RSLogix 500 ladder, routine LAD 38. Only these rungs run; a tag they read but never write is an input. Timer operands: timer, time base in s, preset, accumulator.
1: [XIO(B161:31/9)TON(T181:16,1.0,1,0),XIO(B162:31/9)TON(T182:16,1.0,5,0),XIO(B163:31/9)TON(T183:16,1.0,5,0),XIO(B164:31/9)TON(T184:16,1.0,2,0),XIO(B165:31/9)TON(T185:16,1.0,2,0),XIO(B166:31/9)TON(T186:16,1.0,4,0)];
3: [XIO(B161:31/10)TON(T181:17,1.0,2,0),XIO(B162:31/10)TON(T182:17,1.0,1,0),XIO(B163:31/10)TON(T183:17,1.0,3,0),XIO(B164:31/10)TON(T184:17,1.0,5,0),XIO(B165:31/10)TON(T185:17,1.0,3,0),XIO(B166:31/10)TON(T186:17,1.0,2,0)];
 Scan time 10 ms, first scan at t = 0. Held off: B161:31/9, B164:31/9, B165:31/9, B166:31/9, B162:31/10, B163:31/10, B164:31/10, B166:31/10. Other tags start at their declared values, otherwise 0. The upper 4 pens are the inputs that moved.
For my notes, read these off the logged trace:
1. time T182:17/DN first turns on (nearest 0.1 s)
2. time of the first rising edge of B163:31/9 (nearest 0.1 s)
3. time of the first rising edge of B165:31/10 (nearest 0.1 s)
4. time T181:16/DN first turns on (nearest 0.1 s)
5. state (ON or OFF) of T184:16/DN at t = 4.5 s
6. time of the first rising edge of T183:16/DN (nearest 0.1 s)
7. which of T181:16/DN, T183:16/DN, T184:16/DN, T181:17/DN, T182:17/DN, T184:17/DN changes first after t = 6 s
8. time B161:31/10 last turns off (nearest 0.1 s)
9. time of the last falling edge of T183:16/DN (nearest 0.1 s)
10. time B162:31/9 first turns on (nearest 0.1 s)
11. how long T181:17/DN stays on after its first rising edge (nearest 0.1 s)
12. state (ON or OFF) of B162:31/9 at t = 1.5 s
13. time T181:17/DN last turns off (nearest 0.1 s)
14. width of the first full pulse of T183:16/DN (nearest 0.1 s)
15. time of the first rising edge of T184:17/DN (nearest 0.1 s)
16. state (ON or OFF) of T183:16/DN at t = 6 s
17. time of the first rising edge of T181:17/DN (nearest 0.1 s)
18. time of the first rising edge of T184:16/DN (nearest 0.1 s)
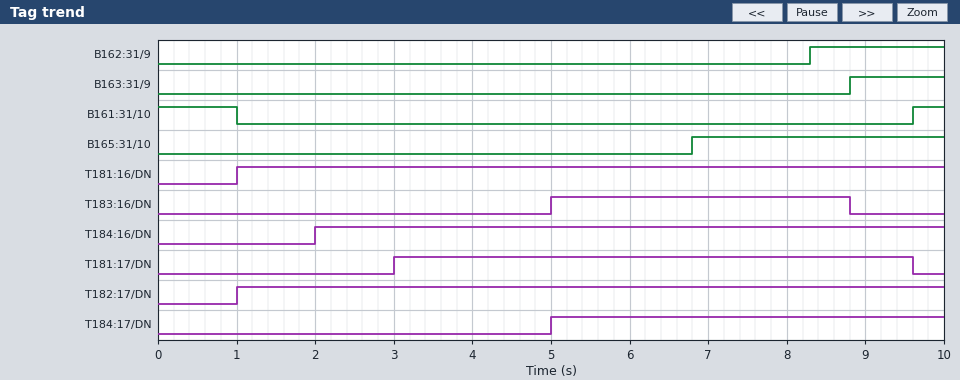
1.0 s
8.8 s
6.8 s
1.0 s
ON
5.0 s
T183:16/DN
1.0 s
8.8 s
8.3 s
6.6 s
OFF
9.6 s
3.8 s
5.0 s
ON
3.0 s
2.0 s
